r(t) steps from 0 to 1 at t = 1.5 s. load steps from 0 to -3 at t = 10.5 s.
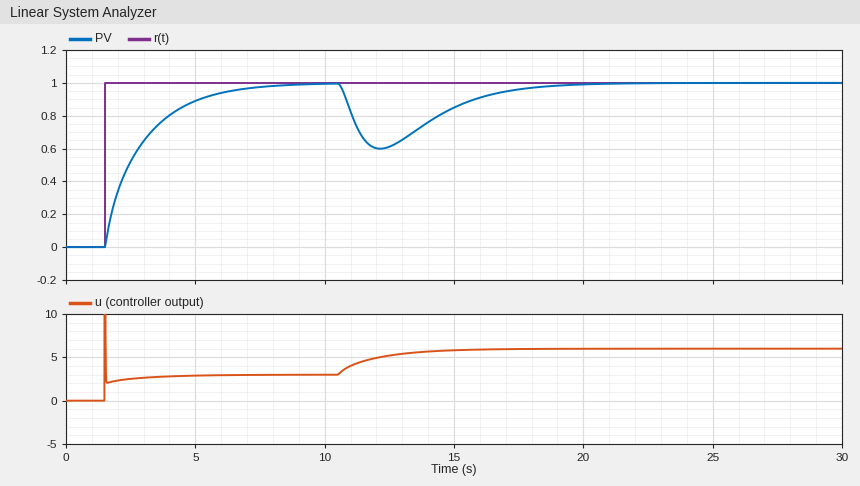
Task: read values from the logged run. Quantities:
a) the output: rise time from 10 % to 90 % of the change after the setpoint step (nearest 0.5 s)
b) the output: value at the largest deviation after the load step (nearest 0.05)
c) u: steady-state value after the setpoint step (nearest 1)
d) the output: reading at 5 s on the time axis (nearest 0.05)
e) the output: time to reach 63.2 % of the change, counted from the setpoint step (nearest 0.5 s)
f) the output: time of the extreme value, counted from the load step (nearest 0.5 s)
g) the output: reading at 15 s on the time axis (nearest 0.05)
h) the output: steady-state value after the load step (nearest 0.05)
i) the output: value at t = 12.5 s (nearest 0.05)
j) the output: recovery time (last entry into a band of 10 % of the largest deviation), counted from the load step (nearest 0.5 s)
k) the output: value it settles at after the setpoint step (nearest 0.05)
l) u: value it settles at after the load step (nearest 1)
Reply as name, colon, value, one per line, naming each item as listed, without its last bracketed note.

the output: rise time from 10 % to 90 % of the change after the setpoint step: 3.5 s
the output: value at the largest deviation after the load step: 0.60
u: steady-state value after the setpoint step: 3
the output: reading at 5 s on the time axis: 0.90
the output: time to reach 63.2 % of the change, counted from the setpoint step: 1.5 s
the output: time of the extreme value, counted from the load step: 1.5 s
the output: reading at 15 s on the time axis: 0.85
the output: steady-state value after the load step: 1.00
the output: value at t = 12.5 s: 0.60
the output: recovery time (last entry into a band of 10 % of the largest deviation), counted from the load step: 7.0 s
the output: value it settles at after the setpoint step: 1.00
u: value it settles at after the load step: 6
